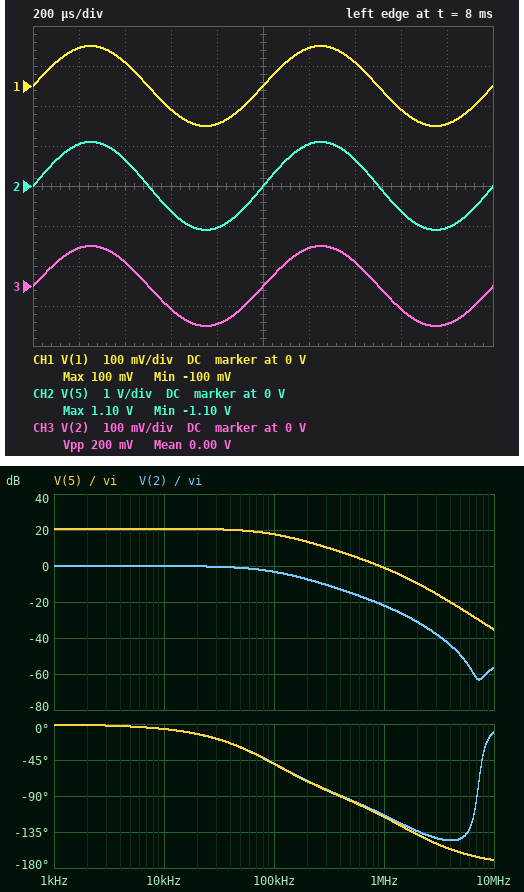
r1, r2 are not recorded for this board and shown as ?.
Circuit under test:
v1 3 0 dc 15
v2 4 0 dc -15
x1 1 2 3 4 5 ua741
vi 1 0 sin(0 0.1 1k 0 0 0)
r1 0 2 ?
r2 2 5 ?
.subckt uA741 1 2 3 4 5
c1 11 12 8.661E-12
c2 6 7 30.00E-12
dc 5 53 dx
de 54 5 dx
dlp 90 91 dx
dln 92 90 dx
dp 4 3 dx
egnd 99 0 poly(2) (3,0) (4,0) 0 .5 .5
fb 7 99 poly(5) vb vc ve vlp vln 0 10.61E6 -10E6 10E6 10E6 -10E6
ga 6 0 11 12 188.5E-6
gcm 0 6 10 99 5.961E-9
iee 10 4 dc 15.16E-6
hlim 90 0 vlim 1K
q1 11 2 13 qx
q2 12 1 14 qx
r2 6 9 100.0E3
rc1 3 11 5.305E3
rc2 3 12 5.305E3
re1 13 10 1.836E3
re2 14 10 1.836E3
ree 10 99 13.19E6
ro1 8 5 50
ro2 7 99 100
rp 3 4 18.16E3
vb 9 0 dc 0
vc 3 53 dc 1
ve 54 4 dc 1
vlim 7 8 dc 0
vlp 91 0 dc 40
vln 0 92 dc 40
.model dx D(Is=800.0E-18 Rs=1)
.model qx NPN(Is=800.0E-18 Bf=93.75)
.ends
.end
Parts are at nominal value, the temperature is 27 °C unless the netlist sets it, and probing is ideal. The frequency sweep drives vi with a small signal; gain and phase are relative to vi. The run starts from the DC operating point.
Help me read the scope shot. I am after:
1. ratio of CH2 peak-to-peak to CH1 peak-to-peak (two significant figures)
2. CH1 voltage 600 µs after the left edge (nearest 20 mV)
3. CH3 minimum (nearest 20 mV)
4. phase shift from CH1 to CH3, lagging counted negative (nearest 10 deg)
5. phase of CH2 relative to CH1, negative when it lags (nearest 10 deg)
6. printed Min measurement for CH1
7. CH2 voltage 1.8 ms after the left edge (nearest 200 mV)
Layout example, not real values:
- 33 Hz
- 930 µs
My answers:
- 11
- -60 mV
- -100 mV
- 0 deg
- 0 deg
- -100 mV
- -1.0 V
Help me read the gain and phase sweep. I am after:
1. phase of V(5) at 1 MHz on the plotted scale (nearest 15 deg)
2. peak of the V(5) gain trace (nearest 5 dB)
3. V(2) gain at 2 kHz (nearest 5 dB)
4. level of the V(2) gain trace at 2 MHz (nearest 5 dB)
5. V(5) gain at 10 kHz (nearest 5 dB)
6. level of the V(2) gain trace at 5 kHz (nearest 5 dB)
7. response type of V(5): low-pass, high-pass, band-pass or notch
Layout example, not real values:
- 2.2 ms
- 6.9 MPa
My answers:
- -120 deg
- 20 dB
- 0 dB
- -30 dB
- 20 dB
- 0 dB
- low-pass
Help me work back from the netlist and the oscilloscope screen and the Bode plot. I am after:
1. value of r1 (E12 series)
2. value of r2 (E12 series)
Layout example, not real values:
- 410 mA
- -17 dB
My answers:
- 3.3 kΩ
- 33 kΩ
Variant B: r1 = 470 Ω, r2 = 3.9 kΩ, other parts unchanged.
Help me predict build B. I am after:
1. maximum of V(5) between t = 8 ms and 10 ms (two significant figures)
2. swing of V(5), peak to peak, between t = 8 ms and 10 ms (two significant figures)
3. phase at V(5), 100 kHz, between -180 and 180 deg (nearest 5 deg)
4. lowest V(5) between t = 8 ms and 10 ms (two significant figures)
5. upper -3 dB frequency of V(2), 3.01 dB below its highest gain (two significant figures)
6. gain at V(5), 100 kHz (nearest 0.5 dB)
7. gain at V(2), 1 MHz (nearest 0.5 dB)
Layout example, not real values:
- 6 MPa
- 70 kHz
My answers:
- 930 mV
- 1.9 V
- -45 deg
- -930 mV
- 110 kHz
- 17.0 dB
- -20.5 dB
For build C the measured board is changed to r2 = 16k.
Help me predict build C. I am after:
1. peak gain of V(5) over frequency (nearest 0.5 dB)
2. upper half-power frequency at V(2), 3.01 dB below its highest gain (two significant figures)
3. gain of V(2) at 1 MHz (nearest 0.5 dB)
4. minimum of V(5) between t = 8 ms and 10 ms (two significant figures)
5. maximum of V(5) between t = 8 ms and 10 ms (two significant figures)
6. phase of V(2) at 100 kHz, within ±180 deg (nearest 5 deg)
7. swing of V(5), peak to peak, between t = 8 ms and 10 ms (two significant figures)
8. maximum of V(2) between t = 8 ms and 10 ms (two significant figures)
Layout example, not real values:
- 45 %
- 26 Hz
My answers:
- 15.5 dB
- 190 kHz
- -16.0 dB
- -580 mV
- 590 mV
- -30 deg
- 1.2 V
- 100 mV
